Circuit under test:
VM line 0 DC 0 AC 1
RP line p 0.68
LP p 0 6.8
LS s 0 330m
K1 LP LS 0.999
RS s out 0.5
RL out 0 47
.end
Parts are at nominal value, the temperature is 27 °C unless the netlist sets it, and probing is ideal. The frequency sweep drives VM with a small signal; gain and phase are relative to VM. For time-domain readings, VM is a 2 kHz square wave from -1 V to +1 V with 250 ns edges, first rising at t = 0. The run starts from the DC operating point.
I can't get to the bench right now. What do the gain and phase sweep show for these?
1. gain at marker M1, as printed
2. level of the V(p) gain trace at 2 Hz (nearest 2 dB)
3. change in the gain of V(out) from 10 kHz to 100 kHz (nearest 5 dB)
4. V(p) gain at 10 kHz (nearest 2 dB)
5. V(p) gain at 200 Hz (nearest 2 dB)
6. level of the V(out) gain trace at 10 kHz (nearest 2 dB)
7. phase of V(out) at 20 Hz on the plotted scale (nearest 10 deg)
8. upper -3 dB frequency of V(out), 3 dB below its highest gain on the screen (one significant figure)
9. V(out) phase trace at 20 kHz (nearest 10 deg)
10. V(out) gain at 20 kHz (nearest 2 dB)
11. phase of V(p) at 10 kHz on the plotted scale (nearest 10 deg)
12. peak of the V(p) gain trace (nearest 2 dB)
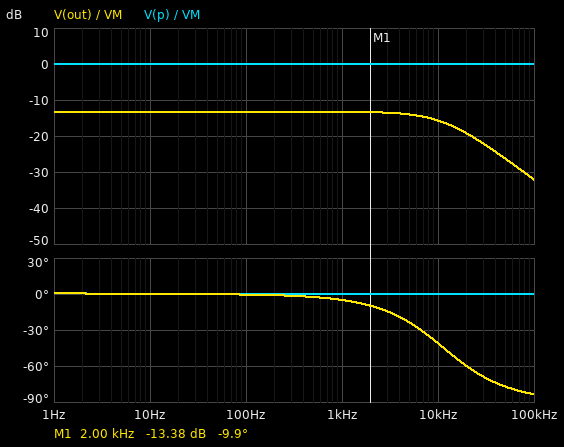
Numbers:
-13.38 dB
0 dB
-15 dB
0 dB
0 dB
-16 dB
0 deg
10 kHz
-60 deg
-20 dB
0 deg
0 dB
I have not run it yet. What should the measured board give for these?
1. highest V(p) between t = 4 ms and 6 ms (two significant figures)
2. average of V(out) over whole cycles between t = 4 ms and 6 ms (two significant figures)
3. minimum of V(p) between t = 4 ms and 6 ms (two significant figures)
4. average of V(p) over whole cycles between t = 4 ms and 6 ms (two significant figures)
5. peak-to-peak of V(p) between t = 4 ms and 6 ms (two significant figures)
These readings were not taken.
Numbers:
2.0 V
220 mV
-2.0 mV
1.0 V
2.0 V
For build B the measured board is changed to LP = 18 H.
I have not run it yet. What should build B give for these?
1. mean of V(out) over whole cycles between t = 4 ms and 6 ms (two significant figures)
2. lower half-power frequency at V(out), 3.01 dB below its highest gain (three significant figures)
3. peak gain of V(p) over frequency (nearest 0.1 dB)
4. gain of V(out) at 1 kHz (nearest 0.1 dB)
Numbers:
130 mV
6.01 mHz
0 dB
-17.5 dB
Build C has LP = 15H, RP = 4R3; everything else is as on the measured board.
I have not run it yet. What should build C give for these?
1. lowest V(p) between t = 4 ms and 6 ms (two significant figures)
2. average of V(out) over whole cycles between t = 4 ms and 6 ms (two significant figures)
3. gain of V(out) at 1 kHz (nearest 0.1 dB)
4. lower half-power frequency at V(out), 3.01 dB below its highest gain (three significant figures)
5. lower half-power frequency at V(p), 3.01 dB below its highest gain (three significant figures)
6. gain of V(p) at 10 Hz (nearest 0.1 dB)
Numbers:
-5.6 mV
150 mV
-16.7 dB
45.5 mHz
45.7 mHz
0 dB
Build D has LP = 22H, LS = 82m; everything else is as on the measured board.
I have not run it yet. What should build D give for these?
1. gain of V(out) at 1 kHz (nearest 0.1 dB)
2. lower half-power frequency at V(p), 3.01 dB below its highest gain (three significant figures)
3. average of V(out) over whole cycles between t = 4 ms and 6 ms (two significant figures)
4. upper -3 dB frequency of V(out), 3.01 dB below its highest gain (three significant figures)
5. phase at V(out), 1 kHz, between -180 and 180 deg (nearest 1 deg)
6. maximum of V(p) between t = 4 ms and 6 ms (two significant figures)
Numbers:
-24.4 dB
4.92 mHz
60 mV
46.1 kHz
-1 deg
2.0 V
